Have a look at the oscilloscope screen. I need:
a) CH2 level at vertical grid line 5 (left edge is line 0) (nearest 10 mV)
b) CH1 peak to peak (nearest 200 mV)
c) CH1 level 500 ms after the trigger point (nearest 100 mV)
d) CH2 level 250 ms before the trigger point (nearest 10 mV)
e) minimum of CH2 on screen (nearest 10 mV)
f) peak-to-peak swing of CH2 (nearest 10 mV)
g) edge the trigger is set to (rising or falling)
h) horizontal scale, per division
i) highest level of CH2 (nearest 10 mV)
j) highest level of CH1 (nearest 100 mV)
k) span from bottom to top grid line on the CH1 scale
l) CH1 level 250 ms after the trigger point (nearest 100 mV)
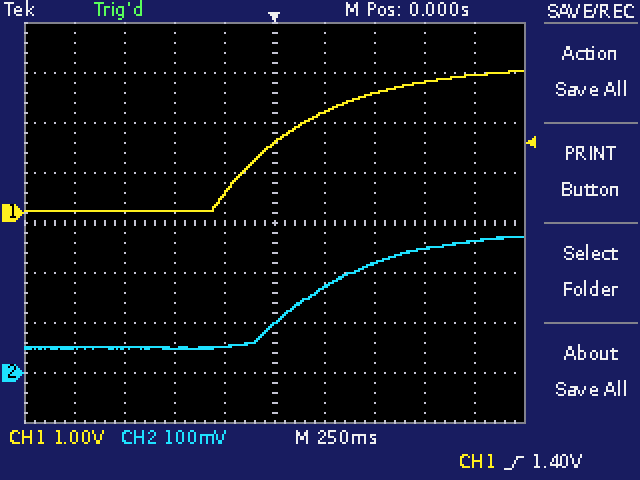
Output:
100 mV
2.8 V
2.4 V
50 mV
50 mV
220 mV
rising
250 ms
270 mV
2.8 V
8 V
2.0 V
